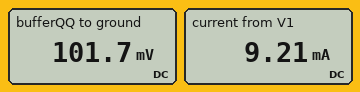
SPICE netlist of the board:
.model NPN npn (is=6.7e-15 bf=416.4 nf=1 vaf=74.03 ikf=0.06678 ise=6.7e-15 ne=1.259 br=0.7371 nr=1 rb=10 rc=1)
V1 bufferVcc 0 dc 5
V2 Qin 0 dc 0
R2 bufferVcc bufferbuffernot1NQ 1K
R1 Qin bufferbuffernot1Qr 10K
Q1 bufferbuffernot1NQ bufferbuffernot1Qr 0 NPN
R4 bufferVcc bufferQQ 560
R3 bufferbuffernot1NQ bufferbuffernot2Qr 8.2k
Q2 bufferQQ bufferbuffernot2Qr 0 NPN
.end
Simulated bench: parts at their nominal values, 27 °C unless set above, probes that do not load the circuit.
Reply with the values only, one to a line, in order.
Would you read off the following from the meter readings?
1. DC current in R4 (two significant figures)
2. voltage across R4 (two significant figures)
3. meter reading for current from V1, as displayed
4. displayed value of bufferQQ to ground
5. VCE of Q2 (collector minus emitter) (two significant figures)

8.7 mA
4.9 V
9.21 mA
101.7 mV
100 mV
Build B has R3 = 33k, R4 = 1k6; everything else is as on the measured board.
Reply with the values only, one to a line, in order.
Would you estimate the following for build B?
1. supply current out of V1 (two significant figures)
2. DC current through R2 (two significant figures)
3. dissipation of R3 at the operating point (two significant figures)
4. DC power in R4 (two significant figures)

3.2 mA
130 µA
530 µW
15 mW
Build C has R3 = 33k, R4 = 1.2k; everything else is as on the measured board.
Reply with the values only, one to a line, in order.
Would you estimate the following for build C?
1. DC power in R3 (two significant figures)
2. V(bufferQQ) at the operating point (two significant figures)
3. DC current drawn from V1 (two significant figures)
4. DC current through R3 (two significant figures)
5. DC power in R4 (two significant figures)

530 µW
110 mV
4.2 mA
130 µA
20 mW
